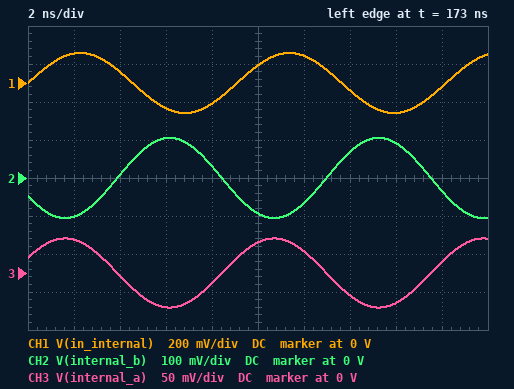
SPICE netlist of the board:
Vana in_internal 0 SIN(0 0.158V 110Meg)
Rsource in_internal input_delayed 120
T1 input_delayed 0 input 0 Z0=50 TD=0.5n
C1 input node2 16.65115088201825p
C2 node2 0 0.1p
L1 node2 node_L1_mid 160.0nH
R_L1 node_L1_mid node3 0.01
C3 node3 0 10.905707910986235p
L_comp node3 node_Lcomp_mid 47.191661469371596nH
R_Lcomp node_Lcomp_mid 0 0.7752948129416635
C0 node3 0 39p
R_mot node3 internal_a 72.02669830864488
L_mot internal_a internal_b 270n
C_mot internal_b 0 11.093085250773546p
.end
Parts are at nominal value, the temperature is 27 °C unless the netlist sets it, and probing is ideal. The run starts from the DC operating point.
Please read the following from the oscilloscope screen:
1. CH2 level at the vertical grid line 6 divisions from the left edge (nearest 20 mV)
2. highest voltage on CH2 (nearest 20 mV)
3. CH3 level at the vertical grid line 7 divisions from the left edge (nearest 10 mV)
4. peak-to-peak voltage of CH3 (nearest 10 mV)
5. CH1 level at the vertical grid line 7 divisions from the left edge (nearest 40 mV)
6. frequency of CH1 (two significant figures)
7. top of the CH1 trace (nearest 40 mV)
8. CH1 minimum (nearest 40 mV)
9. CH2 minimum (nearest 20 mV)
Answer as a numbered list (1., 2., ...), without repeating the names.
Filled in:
1. -60 mV
2. 100 mV
3. -30 mV
4. 90 mV
5. -40 mV
6. 110 MHz
7. 160 mV
8. -160 mV
9. -100 mV
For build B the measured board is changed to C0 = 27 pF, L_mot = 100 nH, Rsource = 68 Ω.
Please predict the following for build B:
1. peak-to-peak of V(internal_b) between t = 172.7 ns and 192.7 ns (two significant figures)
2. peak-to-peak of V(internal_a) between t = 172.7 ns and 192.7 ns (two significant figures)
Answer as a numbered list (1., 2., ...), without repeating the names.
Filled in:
1. 270 mV
2. 130 mV
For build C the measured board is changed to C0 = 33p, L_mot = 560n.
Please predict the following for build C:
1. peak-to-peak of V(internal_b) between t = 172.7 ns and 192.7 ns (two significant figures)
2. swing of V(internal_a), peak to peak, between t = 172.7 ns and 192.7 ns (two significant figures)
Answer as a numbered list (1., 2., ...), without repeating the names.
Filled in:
1. 110 mV
2. 220 mV
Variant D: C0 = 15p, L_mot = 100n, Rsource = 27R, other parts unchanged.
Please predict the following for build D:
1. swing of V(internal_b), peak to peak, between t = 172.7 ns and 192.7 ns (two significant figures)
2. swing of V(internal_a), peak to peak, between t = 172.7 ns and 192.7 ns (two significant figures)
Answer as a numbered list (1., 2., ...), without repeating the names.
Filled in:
1. 310 mV
2. 140 mV
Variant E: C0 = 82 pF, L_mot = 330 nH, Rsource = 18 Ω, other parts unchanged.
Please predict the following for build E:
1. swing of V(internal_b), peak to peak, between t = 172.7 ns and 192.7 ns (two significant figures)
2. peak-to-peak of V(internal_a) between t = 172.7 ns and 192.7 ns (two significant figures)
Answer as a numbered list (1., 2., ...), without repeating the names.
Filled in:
1. 470 mV
2. 350 mV
